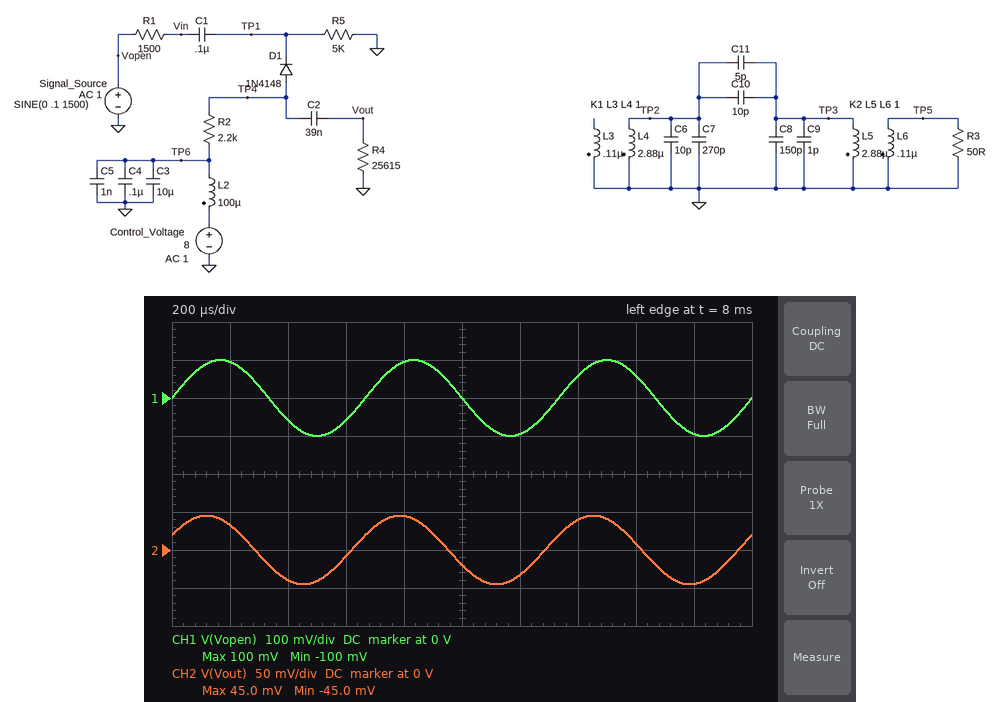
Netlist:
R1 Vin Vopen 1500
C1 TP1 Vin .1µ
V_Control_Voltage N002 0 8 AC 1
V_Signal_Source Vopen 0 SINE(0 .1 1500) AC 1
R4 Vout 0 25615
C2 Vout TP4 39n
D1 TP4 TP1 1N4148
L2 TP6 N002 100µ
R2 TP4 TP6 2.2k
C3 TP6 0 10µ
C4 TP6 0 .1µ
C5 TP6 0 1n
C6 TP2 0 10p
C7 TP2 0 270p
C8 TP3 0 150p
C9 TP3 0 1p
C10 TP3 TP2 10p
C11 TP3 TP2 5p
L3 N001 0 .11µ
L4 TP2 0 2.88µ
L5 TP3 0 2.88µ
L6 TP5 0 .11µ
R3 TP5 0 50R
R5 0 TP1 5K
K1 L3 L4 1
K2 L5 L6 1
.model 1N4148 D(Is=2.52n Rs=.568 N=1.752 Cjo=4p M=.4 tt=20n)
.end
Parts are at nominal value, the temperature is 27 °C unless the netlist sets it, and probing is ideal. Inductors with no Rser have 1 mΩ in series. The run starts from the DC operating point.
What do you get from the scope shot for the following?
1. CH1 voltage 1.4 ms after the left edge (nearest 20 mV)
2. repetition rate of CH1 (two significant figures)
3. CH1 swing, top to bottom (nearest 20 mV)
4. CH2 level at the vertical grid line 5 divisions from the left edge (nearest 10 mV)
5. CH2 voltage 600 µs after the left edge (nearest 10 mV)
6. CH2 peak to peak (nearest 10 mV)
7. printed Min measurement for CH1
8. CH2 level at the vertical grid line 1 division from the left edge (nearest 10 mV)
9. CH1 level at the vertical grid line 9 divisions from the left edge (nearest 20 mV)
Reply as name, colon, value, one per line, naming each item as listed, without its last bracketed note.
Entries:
CH1 voltage 1.4 ms after the left edge: 60 mV
repetition rate of CH1: 1.5 kHz
CH1 swing, top to bottom: 200 mV
CH2 level at the vertical grid line 5 divisions from the left edge: -20 mV
CH2 voltage 600 µs after the left edge: -10 mV
CH2 peak to peak: 90 mV
printed Min measurement for CH1: -100 mV
CH2 level at the vertical grid line 1 division from the left edge: 30 mV
CH1 level at the vertical grid line 9 divisions from the left edge: -100 mV
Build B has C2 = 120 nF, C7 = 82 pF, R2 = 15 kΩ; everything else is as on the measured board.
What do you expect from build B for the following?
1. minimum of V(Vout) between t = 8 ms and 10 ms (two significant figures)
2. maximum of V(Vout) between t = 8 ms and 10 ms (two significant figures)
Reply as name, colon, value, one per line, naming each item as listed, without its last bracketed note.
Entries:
minimum of V(Vout) between t = 8 ms and 10 ms: -66 mV
maximum of V(Vout) between t = 8 ms and 10 ms: 66 mV
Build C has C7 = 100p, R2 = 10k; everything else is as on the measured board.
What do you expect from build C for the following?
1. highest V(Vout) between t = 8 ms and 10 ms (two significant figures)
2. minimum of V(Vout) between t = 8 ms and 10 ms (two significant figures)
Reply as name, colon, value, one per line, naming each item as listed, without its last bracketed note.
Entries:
highest V(Vout) between t = 8 ms and 10 ms: 63 mV
minimum of V(Vout) between t = 8 ms and 10 ms: -63 mV
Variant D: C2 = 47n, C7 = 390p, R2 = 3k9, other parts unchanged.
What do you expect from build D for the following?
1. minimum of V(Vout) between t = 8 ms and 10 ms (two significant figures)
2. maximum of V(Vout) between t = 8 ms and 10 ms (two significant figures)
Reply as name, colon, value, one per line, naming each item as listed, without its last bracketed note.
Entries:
minimum of V(Vout) between t = 8 ms and 10 ms: -54 mV
maximum of V(Vout) between t = 8 ms and 10 ms: 54 mV
